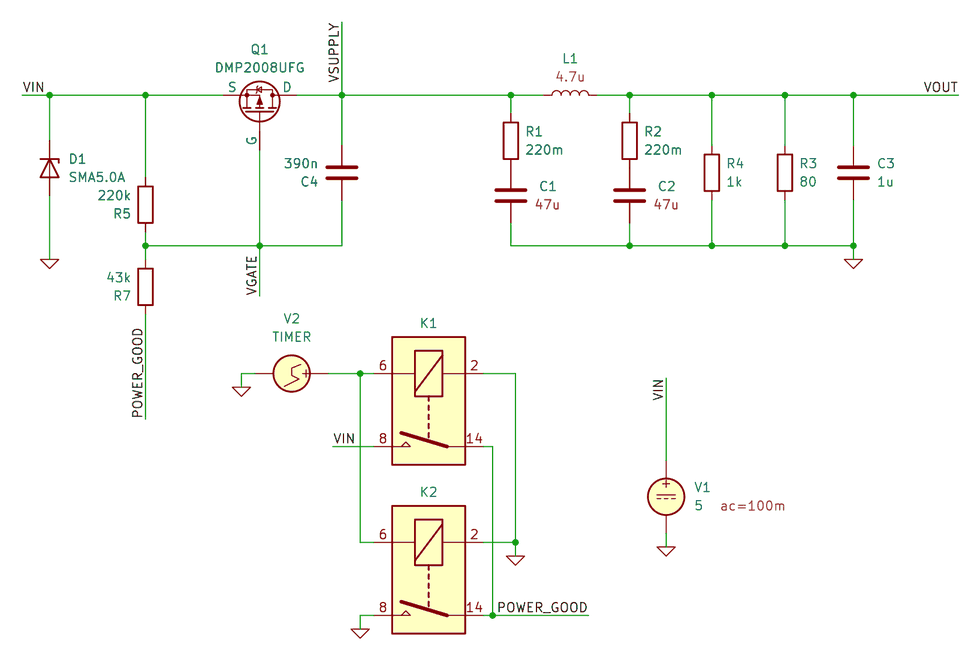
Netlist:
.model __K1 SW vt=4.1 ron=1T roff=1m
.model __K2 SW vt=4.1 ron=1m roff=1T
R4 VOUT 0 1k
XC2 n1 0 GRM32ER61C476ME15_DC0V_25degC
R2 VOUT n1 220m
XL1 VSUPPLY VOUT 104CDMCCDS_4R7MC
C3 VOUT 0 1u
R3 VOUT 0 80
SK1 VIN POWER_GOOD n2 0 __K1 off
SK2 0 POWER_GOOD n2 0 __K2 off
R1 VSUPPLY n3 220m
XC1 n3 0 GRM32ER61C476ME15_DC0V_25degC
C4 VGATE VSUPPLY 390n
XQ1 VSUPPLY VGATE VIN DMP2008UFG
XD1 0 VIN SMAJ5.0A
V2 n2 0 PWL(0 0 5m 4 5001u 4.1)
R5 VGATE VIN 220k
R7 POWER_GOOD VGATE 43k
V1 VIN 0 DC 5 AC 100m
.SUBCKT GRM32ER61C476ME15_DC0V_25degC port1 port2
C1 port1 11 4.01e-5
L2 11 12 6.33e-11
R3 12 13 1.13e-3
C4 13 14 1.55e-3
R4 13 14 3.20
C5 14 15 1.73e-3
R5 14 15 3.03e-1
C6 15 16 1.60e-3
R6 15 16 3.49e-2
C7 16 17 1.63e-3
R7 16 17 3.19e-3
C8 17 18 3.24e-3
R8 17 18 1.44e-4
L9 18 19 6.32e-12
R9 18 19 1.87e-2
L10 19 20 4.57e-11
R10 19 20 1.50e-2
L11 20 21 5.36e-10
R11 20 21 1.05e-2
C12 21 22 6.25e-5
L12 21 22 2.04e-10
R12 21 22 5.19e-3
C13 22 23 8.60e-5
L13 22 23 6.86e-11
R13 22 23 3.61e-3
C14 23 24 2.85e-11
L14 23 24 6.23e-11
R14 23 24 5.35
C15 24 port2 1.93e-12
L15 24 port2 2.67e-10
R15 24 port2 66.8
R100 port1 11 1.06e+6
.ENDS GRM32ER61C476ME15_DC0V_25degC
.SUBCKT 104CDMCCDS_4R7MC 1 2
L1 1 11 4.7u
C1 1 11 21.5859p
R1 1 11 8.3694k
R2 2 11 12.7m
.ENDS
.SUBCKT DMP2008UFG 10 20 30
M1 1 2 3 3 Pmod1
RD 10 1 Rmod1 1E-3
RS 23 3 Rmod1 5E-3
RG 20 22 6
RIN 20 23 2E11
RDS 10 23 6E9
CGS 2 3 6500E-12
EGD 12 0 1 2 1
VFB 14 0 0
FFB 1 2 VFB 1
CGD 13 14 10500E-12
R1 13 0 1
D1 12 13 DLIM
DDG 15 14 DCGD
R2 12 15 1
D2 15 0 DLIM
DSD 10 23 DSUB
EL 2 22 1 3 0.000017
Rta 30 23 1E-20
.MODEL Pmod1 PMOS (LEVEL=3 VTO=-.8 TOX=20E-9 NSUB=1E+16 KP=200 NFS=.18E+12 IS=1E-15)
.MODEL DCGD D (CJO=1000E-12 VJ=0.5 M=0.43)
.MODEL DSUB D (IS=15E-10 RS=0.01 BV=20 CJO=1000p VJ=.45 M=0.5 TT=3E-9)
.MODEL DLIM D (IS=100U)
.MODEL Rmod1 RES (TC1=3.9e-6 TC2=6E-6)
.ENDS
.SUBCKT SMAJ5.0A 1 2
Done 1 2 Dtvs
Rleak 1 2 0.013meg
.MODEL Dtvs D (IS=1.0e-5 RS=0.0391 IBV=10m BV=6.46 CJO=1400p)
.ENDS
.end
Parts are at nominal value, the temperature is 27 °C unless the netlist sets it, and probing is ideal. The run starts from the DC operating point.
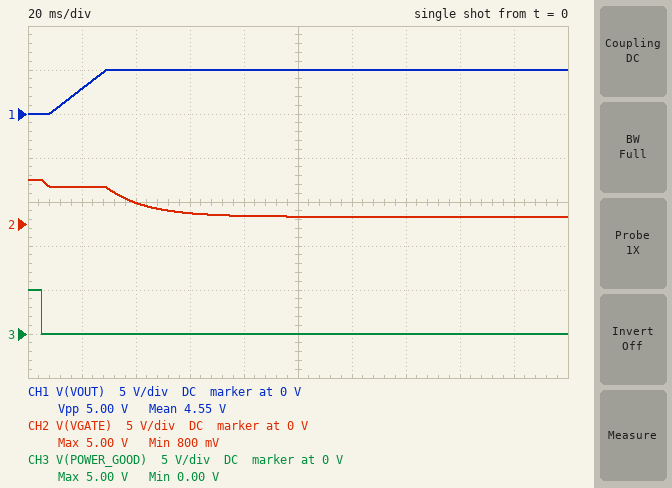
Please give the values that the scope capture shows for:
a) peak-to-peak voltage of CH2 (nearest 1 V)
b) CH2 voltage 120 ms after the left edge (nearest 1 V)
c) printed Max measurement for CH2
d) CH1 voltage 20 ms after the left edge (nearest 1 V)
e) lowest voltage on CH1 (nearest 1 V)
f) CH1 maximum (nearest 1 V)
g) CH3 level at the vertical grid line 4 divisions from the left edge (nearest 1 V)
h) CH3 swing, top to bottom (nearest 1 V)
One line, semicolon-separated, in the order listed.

4 V; 1 V; 5.00 V; 3 V; 0 V; 5 V; 0 V; 5 V
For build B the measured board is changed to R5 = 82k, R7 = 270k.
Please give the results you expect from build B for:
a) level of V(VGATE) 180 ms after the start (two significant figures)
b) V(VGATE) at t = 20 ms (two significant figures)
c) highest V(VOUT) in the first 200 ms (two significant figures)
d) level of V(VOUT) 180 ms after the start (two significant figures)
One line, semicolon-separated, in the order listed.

4.2 V; 4.5 V; 2.7 V; 2.4 V
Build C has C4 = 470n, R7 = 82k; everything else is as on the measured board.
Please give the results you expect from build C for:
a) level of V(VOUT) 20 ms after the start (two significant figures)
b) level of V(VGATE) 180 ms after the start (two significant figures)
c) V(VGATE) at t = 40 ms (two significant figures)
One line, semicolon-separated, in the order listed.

840 mV; 1.4 V; 4.2 V
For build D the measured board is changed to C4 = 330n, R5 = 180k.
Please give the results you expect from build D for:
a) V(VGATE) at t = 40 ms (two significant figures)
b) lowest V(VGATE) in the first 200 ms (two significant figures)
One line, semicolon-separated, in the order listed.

1.9 V; 960 mV
